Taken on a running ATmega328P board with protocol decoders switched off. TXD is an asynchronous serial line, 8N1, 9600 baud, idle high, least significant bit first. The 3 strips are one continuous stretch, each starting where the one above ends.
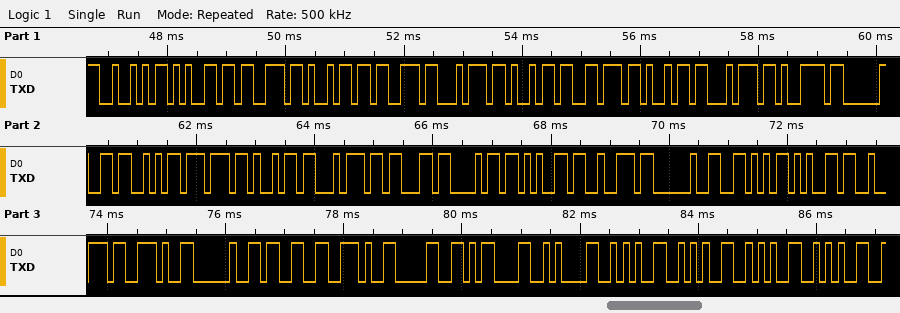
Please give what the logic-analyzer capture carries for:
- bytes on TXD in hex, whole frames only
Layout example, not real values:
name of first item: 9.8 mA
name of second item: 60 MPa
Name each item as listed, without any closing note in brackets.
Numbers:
bytes on TXD in hex, whole frames only: 52 65 73 69 73 74 69 76 69 74 79 20 53 77 69 74 63 68 65 72 20 56 65 72 2E 20 33 2E 30 0D 0A 2A 2A 2A 2A
